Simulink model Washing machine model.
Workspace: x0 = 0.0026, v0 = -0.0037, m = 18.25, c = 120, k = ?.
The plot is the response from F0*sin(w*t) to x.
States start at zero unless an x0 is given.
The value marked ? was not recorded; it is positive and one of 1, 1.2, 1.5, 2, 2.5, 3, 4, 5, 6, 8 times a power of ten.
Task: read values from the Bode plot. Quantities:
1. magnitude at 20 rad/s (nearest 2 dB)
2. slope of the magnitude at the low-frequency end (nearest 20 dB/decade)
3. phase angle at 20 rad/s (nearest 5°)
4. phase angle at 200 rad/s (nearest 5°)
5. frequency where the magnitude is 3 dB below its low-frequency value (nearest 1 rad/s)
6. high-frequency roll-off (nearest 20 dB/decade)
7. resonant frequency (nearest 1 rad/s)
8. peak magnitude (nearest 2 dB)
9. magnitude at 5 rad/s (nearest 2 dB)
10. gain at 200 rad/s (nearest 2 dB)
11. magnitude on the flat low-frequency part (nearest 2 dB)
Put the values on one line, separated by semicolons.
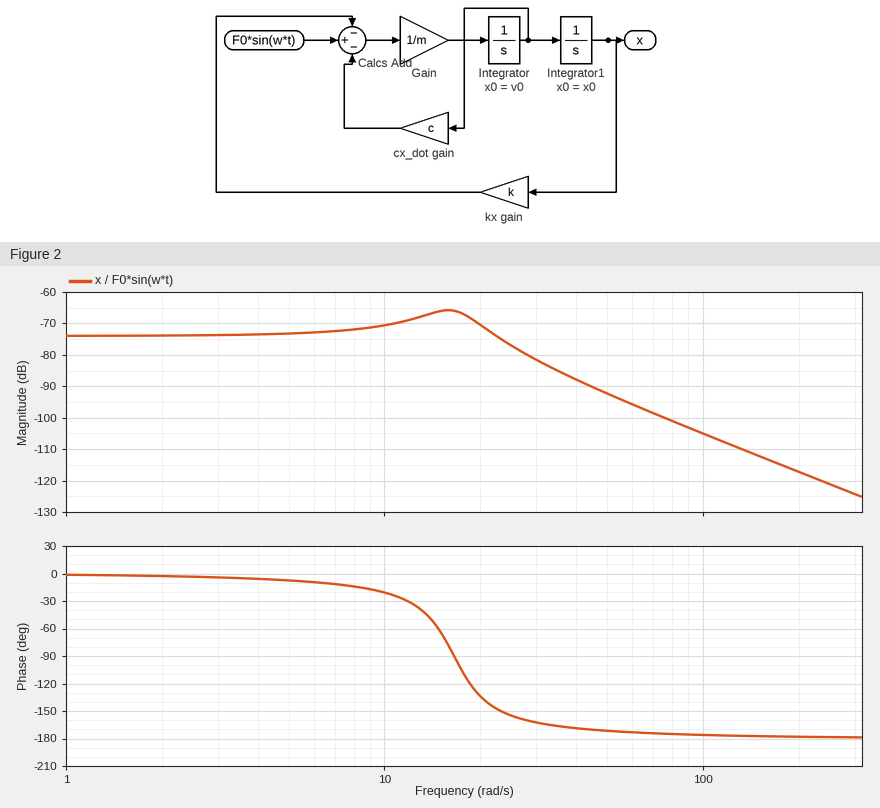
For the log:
-70 dB; 0 dB/decade; -135°; -180°; 25 rad/s; -40 dB/decade; 16 rad/s; -66 dB; -74 dB; -118 dB; -74 dB
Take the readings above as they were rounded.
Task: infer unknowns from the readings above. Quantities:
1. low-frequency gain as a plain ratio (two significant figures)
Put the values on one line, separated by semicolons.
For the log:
0.00020
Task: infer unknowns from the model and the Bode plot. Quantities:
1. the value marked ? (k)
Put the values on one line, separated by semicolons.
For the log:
5000
